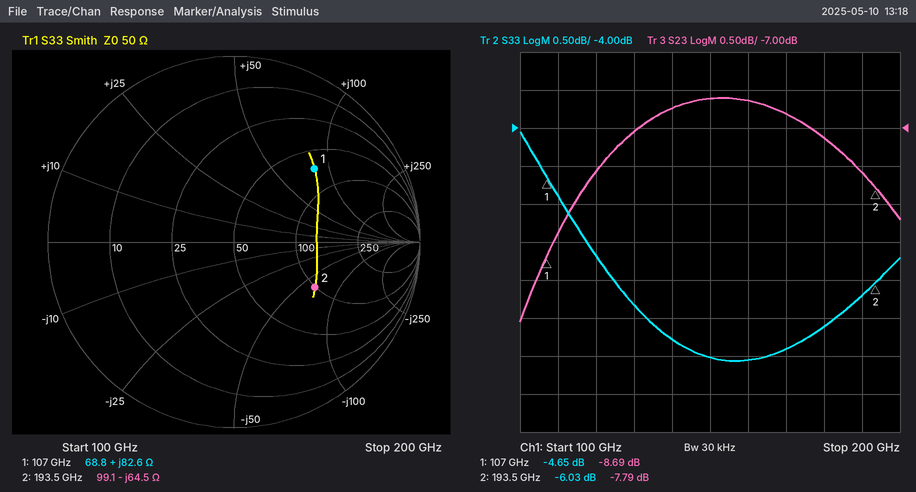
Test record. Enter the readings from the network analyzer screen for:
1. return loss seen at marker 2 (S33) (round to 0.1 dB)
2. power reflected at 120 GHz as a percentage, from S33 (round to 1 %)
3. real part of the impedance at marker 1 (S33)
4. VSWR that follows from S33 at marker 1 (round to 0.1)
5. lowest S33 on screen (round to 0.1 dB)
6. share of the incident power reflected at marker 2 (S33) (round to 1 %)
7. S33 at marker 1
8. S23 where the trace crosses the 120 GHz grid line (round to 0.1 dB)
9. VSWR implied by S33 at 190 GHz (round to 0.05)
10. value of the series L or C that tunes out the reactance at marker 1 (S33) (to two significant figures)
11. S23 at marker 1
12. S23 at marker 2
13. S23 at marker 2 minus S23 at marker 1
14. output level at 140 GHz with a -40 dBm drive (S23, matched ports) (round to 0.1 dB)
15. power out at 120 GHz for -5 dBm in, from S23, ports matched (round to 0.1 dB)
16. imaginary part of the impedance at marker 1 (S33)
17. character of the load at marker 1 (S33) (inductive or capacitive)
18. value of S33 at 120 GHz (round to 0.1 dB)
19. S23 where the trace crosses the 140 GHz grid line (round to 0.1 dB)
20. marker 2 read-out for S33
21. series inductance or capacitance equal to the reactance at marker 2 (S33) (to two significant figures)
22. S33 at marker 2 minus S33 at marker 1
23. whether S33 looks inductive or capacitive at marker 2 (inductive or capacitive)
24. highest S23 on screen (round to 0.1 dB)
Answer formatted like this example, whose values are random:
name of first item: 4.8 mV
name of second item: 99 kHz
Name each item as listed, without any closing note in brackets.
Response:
return loss seen at marker 2 (S33): 6.0 dB
power reflected at 120 GHz as a percentage, from S33: 27 %
real part of the impedance at marker 1: 68.8 Ω
VSWR that follows from S33 at marker 1: 3.8
lowest S33 on screen: -7.1 dB
share of the incident power reflected at marker 2 (S33): 25 %
S33 at marker 1: -4.65 dB
S23 where the trace crosses the 120 GHz grid line: -7.6 dB
VSWR implied by S33 at 190 GHz: 2.90
value of the series L or C that tunes out the reactance at marker 1 (S33): 18 fF
S23 at marker 1: -8.69 dB
S23 at marker 2: -7.79 dB
S23 at marker 2 minus S23 at marker 1: 0.90 dB
output level at 140 GHz with a -40 dBm drive (S23, matched ports): -46.7 dBm
power out at 120 GHz for -5 dBm in, from S23, ports matched: -12.6 dBm
imaginary part of the impedance at marker 1: +82.6 Ω
character of the load at marker 1 (S33): inductive
value of S33 at 120 GHz: -5.7 dB
S23 where the trace crosses the 140 GHz grid line: -6.7 dB
marker 2 read-out for S33: -6.03 dB
series inductance or capacitance equal to the reactance at marker 2 (S33): 13 fF
S33 at marker 2 minus S33 at marker 1: -1.38 dB
whether S33 looks inductive or capacitive at marker 2: capacitive
highest S23 on screen: -6.6 dB
